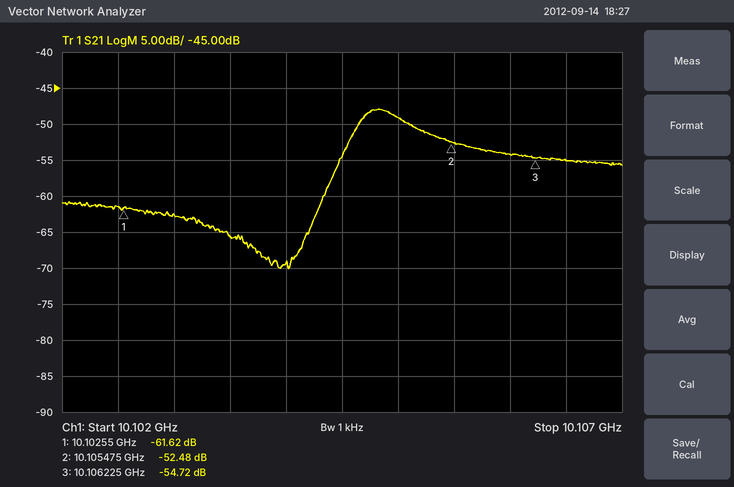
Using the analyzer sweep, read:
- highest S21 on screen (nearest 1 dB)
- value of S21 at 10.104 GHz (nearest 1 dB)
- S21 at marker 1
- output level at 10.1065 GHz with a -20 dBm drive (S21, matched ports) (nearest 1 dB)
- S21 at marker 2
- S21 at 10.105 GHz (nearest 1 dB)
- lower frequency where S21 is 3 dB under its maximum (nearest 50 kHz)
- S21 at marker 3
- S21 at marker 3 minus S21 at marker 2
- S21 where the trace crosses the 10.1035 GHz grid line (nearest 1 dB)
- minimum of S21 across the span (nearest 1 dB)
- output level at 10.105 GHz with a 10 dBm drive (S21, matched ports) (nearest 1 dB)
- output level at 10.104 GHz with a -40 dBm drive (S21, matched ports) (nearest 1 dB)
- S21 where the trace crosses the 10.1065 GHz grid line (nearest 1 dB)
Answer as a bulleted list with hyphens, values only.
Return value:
- -48 dB
- -69 dB
- -61.62 dB
- -75 dBm
- -52.48 dB
- -49 dB
- 10.10460 GHz
- -54.72 dB
- -2.24 dB
- -66 dB
- -70 dB
- -39 dBm
- -109 dBm
- -55 dB
